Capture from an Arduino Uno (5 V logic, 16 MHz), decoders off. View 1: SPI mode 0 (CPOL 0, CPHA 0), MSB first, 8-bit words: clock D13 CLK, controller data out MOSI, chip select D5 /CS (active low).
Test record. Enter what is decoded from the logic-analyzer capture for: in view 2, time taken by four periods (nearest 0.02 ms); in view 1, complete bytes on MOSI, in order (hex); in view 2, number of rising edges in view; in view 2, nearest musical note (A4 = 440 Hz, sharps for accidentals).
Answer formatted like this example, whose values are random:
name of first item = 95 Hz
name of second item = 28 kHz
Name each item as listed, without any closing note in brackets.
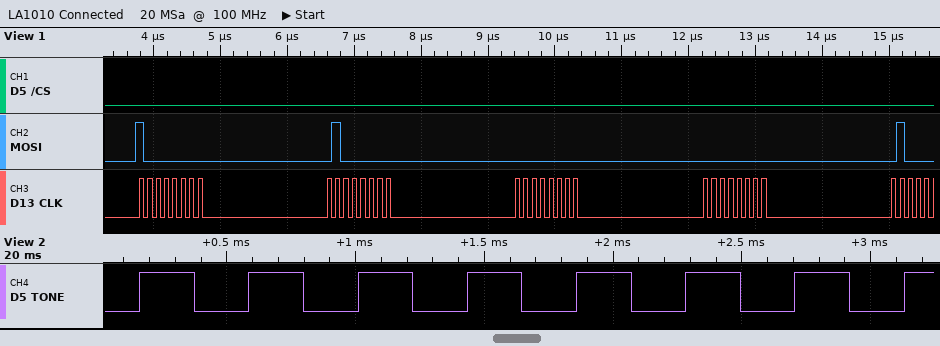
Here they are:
in view 2, time taken by four periods = 1.70 ms
in view 1, complete bytes on MOSI, in order = 0x80 0x40 0x00 0x00
in view 2, number of rising edges in view = 8
in view 2, nearest musical note = D7
